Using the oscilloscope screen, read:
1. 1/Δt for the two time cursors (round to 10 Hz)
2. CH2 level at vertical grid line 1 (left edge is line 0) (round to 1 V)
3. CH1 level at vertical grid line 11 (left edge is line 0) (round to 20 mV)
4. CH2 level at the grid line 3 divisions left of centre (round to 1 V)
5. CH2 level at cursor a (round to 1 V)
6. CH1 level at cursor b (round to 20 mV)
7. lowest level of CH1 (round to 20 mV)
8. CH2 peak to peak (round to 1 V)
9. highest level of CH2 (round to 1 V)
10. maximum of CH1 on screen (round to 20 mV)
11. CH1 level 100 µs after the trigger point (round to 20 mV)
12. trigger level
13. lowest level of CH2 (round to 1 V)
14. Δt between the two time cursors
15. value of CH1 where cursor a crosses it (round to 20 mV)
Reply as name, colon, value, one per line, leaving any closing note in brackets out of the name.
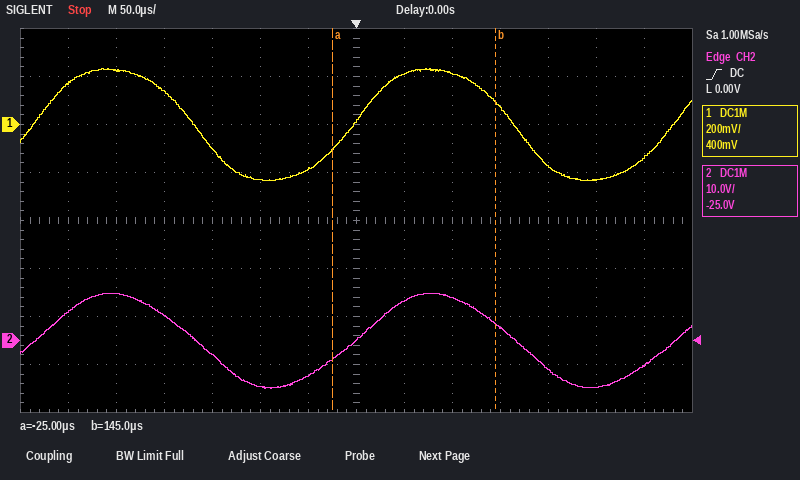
1/Δt for the two time cursors: 5.88 kHz
CH2 level at vertical grid line 1 (left edge is line 0): 6 V
CH1 level at vertical grid line 11 (left edge is line 0): -180 mV
CH2 level at the grid line 3 divisions left of centre: -3 V
CH2 level at cursor a: -4 V
CH1 level at cursor b: 100 mV
lowest level of CH1: -240 mV
CH2 peak to peak: 20 V
highest level of CH2: 10 V
maximum of CH1 on screen: 240 mV
CH1 level 100 µs after the trigger point: 220 mV
trigger level: 0.00 V
lowest level of CH2: -10 V
Δt between the two time cursors: 170 µs
value of CH1 where cursor a crosses it: -100 mV
